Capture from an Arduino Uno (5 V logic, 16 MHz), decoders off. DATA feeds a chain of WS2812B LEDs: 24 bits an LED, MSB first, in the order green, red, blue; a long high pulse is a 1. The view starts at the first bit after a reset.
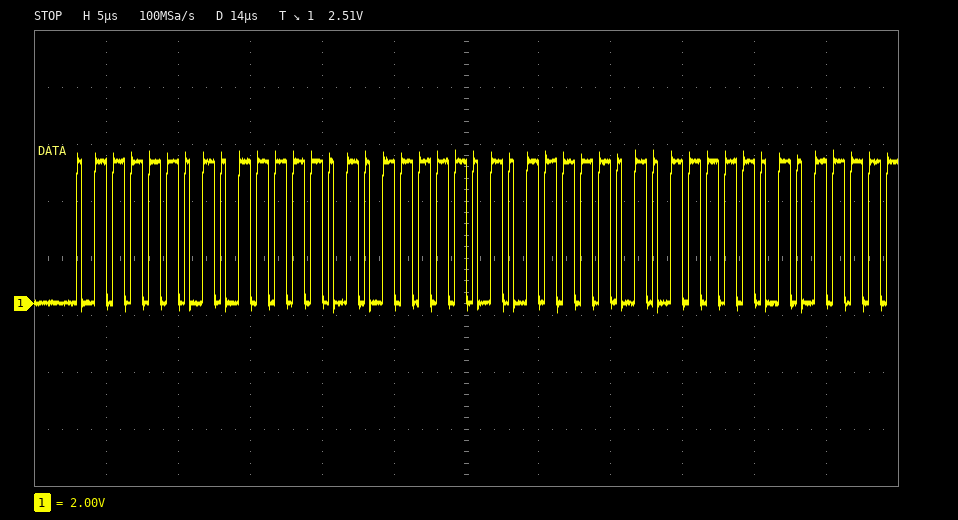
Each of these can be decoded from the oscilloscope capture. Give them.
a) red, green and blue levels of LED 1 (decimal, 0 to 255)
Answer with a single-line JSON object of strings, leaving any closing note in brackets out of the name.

{"red, green and blue levels of LED 1": "125, 125, 125"}
